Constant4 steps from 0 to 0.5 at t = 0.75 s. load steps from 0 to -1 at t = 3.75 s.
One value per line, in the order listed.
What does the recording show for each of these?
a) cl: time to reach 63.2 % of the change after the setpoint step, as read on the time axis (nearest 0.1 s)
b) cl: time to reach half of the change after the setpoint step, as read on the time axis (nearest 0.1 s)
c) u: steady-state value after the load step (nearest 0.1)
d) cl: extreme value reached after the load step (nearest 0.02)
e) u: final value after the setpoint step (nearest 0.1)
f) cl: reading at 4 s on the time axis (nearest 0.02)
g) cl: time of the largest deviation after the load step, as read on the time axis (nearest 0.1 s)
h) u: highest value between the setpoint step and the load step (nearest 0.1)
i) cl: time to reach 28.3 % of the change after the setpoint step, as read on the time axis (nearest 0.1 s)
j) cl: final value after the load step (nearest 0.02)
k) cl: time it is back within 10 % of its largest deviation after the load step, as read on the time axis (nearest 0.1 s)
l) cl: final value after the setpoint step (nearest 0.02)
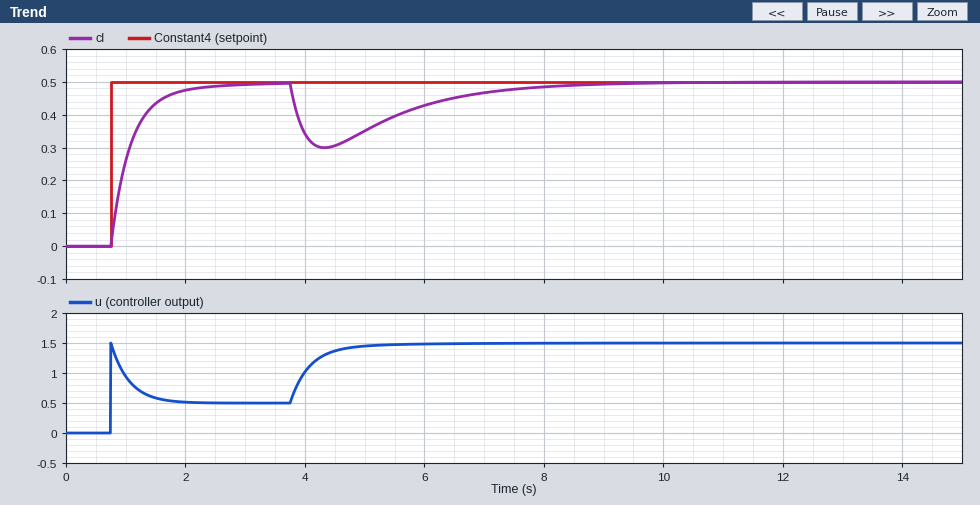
1.1 s
1.0 s
1.5
0.30
0.5
0.34
4.3 s
1.5
0.9 s
0.50
7.7 s
0.50
